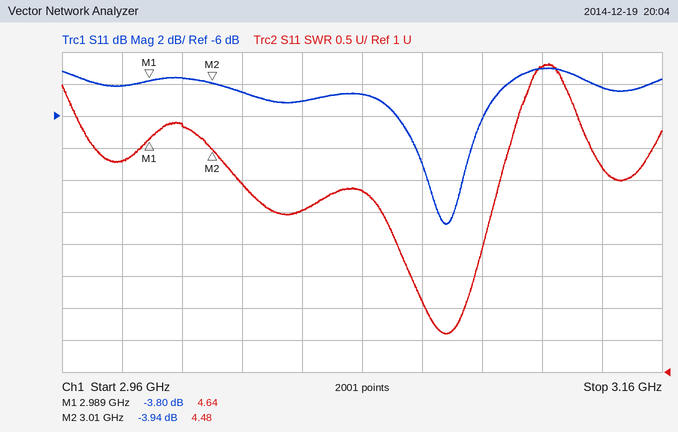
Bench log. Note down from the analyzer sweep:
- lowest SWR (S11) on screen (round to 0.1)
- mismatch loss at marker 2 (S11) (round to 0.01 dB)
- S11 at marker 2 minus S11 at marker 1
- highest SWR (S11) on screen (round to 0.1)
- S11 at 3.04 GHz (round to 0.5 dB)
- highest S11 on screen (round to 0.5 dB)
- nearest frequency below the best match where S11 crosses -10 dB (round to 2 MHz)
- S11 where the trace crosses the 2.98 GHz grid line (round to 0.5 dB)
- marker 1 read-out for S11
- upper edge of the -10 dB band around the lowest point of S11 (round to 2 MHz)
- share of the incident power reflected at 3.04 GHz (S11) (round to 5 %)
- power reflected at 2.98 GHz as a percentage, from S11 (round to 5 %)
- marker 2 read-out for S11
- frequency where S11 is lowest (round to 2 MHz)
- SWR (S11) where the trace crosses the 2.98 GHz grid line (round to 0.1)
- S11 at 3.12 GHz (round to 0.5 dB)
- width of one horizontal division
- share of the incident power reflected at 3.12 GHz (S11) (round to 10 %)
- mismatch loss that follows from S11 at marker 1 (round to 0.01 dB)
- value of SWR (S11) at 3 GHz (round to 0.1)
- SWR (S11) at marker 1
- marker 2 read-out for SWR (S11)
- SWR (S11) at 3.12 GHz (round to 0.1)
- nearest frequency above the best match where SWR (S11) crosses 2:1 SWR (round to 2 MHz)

1.6
2.24 dB
-0.14 dB
5.8
-5.0 dB
-3.0 dB
3.082 GHz
-4.0 dB
-3.80 dB
3.094 GHz
30 %
40 %
-3.94 dB
3.088 GHz
4.3
-3.0 dB
20 MHz
50 %
2.34 dB
4.9
4.64
4.48
5.8
3.094 GHz
